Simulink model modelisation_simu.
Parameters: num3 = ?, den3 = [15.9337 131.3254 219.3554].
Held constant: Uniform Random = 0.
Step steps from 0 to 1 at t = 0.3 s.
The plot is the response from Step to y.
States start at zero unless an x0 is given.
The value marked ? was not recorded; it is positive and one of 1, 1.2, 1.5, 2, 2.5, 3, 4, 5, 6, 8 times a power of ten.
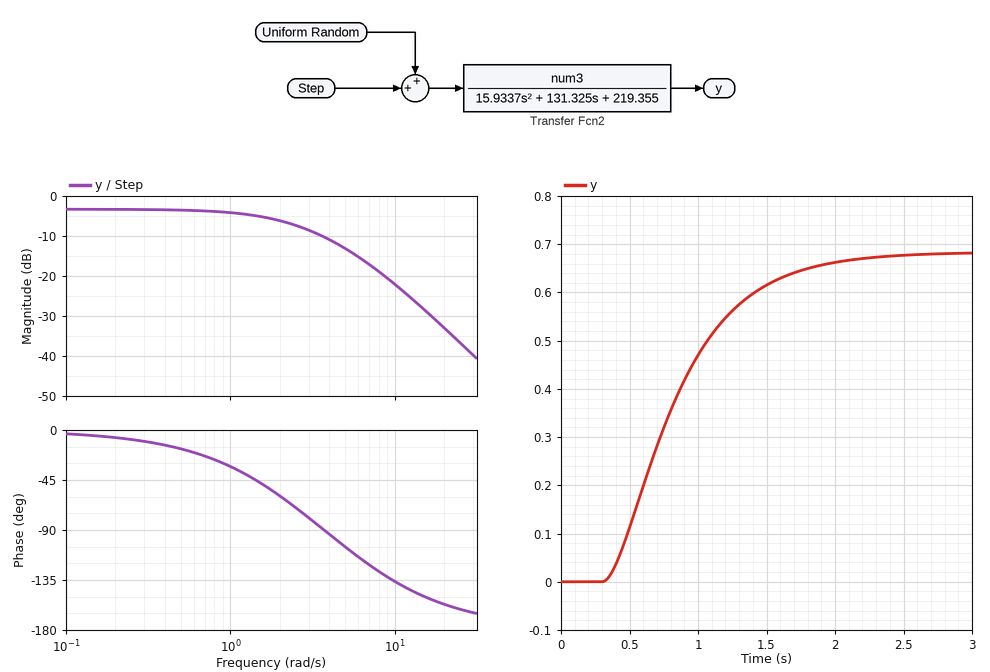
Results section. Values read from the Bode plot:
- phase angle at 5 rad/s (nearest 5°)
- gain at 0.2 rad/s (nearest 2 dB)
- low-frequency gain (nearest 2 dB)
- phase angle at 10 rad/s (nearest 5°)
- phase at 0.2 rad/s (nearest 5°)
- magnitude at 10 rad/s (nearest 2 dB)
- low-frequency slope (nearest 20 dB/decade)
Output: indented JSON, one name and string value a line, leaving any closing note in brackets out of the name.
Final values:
{
  "phase angle at 5 rad/s": "-105°",
  "gain at 0.2 rad/s": "-4 dB",
  "low-frequency gain": "-4 dB",
  "phase angle at 10 rad/s": "-135°",
  "phase at 0.2 rad/s": "-5°",
  "magnitude at 10 rad/s": "-22 dB",
  "low-frequency slope": "0 dB/decade"
}
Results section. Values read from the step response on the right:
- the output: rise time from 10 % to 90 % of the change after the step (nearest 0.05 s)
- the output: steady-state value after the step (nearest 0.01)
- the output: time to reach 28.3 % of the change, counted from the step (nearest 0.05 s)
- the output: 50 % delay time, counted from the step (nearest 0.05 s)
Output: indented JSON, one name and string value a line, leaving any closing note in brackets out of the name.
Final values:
{
  "the output: rise time from 10 % to 90 % of the change after the step": "1.05 s",
  "the output: steady-state value after the step": "0.68",
  "the output: time to reach 28.3 % of the change, counted from the step": "0.30 s",
  "the output: 50 % delay time, counted from the step": "0.50 s"
}
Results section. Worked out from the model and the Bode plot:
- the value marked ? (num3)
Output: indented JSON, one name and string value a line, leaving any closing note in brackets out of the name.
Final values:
{
  "the value marked ?": "150"
}
